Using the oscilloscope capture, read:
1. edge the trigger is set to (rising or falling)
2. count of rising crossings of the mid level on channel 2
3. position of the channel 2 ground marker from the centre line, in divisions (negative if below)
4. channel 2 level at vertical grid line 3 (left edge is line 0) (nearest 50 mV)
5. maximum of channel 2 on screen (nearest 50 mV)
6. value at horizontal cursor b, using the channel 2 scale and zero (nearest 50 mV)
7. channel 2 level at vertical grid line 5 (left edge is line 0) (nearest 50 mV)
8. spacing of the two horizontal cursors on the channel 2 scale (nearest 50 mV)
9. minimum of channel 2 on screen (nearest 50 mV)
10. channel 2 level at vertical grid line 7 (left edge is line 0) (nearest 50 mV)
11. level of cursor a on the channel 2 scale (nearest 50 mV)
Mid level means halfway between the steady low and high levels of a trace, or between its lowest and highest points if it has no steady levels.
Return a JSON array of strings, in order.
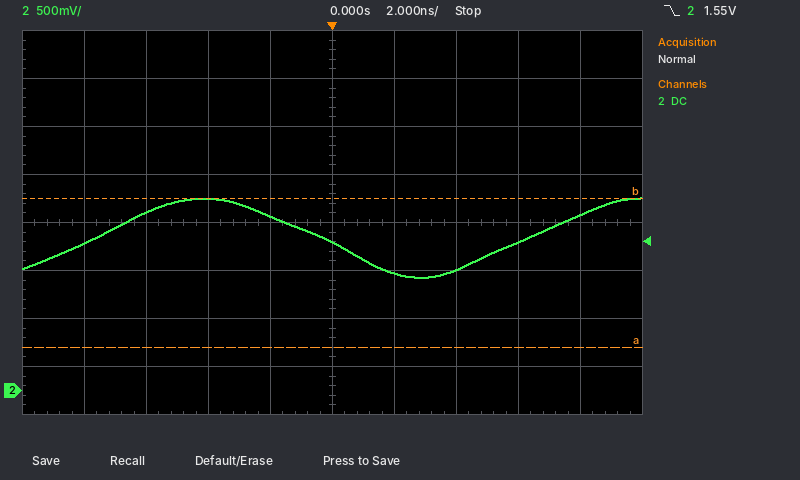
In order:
["falling", "2", "-3.5 div", "2.00 V", "2.00 V", "2.00 V", "1.55 V", "1.55 V", "1.20 V", "1.25 V", "450 mV"]
